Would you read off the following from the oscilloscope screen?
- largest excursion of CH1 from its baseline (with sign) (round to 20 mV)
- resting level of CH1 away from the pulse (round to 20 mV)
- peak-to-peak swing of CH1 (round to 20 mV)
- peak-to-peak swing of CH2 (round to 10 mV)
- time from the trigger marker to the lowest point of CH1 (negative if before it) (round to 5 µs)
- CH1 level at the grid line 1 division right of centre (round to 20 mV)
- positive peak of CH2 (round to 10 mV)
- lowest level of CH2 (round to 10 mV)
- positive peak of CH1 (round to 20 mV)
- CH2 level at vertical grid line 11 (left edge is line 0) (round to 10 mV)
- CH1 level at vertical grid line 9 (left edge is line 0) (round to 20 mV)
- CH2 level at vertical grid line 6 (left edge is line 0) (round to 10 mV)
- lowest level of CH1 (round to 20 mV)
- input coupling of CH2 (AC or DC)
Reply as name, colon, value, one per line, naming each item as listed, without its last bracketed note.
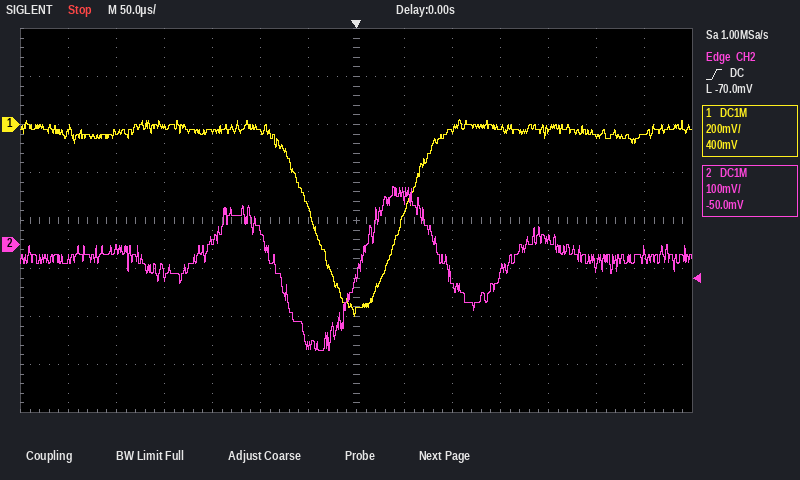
largest excursion of CH1 from its baseline (with sign): -780 mV
resting level of CH1 away from the pulse: -20 mV
peak-to-peak swing of CH1: 820 mV
peak-to-peak swing of CH2: 340 mV
time from the trigger marker to the lowest point of CH1 (negative if before it): 0 µs
CH1 level at the grid line 1 division right of centre: -360 mV
positive peak of CH2: 120 mV
lowest level of CH2: -220 mV
positive peak of CH1: 20 mV
CH2 level at vertical grid line 11 (left edge is line 0): 10 mV
CH1 level at vertical grid line 9 (left edge is line 0): -20 mV
CH2 level at vertical grid line 6 (left edge is line 0): -210 mV
lowest level of CH1: -800 mV
input coupling of CH2: DC
